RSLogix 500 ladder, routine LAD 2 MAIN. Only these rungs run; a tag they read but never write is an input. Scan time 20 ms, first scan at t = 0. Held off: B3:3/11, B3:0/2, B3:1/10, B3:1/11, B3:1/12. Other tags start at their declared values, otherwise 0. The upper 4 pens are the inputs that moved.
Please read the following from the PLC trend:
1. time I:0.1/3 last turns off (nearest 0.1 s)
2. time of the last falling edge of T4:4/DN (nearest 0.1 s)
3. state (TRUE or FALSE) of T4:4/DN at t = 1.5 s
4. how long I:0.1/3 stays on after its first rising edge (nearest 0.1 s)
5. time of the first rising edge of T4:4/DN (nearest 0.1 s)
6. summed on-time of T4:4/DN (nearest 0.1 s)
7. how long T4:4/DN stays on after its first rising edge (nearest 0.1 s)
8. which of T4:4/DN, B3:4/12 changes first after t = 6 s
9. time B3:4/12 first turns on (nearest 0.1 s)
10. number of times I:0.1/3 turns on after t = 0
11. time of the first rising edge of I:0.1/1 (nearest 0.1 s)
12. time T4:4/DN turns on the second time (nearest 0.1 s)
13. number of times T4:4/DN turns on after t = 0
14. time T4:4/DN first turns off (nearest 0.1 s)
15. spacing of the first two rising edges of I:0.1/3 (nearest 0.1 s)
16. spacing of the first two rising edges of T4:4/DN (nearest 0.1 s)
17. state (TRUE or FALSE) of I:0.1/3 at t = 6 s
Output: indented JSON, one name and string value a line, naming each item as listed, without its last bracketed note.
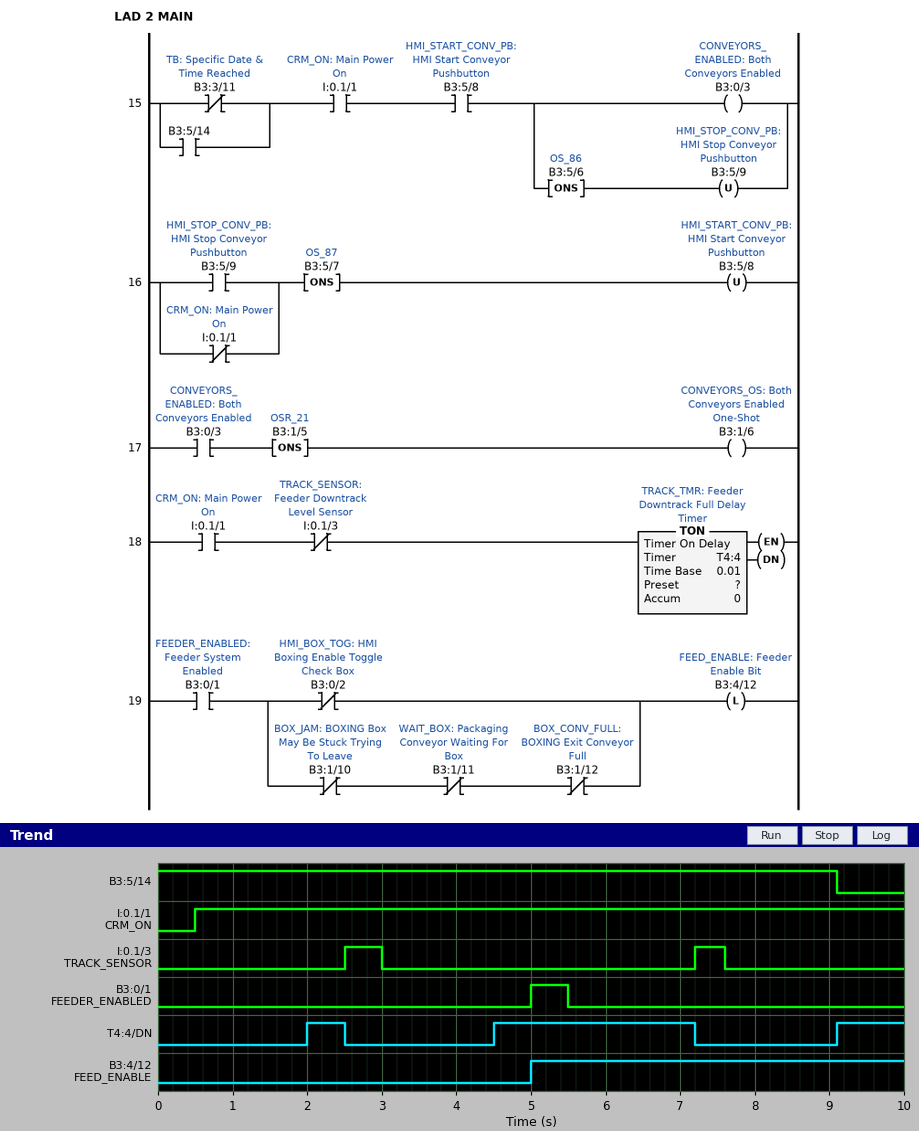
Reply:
{
  "time I:0.1/3 last turns off": "7.6 s",
  "time of the last falling edge of T4:4/DN": "7.2 s",
  "state (TRUE or FALSE) of T4:4/DN at t = 1.5 s": "FALSE",
  "how long I:0.1/3 stays on after its first rising edge": "0.5 s",
  "time of the first rising edge of T4:4/DN": "2.0 s",
  "summed on-time of T4:4/DN": "4.1 s",
  "how long T4:4/DN stays on after its first rising edge": "0.5 s",
  "which of T4:4/DN, B3:4/12 changes first after t = 6 s": "T4:4/DN",
  "time B3:4/12 first turns on": "5.0 s",
  "number of times I:0.1/3 turns on after t = 0": "2",
  "time of the first rising edge of I:0.1/1": "0.5 s",
  "time T4:4/DN turns on the second time": "4.5 s",
  "number of times T4:4/DN turns on after t = 0": "3",
  "time T4:4/DN first turns off": "2.5 s",
  "spacing of the first two rising edges of I:0.1/3": "4.7 s",
  "spacing of the first two rising edges of T4:4/DN": "2.5 s",
  "state (TRUE or FALSE) of I:0.1/3 at t = 6 s": "FALSE"
}
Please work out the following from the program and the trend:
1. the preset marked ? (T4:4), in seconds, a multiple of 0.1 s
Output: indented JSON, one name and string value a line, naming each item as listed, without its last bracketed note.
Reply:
{
  "the preset marked ? (T4:4), in seconds, a multiple of 0.1 s": "1.5 s"
}
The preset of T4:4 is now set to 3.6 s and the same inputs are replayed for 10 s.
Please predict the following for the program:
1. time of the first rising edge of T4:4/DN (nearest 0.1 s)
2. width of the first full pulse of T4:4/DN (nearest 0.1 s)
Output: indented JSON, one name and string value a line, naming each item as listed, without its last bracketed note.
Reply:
{
  "time of the first rising edge of T4:4/DN": "6.6 s",
  "width of the first full pulse of T4:4/DN": "0.6 s"
}
